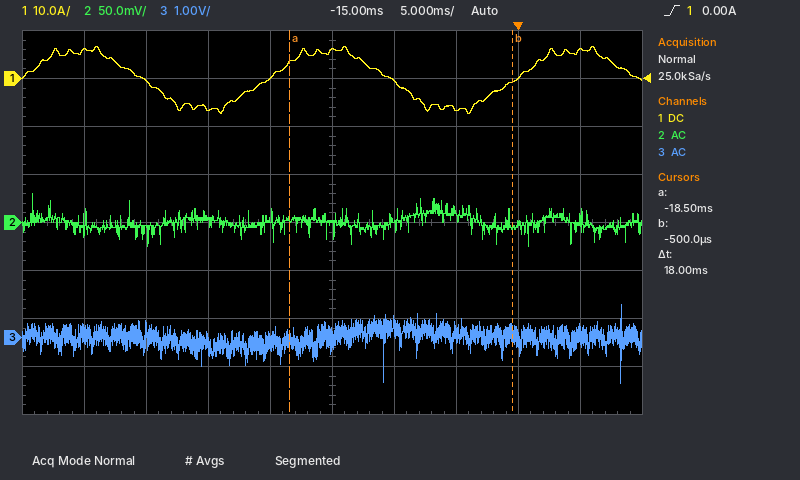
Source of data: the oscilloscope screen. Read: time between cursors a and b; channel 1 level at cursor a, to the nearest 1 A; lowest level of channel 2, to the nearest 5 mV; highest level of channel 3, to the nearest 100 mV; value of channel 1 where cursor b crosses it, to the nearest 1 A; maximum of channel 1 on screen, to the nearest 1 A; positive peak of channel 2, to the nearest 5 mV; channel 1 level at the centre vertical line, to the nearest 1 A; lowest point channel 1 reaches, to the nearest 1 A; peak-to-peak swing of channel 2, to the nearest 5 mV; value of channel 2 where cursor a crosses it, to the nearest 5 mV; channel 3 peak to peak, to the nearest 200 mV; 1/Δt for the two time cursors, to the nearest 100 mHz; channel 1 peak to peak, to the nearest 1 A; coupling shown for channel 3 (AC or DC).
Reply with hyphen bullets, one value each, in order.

- 18 ms
- 3 A
- -25 mV
- 700 mV
- -1 A
- 7 A
- 30 mV
- 6 A
- -7 A
- 55 mV
- 5 mV
- 1.6 V
- 55.6 Hz
- 14 A
- AC
